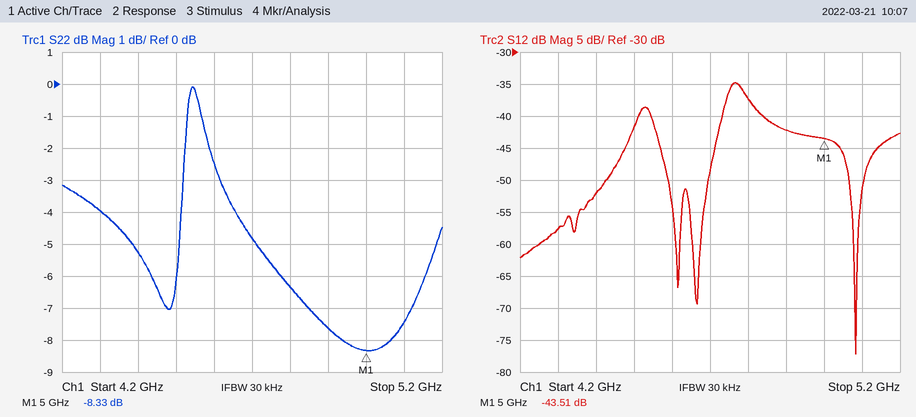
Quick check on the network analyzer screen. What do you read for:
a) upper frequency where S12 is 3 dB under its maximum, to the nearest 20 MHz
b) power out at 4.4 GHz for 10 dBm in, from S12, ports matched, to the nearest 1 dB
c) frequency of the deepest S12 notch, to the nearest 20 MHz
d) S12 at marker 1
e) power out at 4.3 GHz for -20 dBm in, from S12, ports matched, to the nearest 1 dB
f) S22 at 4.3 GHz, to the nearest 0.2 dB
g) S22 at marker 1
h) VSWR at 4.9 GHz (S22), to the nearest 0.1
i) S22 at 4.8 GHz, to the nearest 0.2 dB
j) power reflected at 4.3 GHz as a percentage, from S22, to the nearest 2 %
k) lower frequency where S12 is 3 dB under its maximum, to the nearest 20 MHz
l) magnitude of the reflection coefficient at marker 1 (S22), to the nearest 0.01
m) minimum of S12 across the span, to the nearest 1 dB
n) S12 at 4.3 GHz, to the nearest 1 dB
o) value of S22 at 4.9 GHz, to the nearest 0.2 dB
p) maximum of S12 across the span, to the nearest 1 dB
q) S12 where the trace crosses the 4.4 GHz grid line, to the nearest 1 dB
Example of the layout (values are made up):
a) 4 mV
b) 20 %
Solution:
a) 4.80 GHz
b) -42 dBm
c) 5.08 GHz
d) -43.51 dB
e) -78 dBm
f) -4.0 dB
g) -8.33 dB
h) 2.4
i) -6.4 dB
j) 40 %
k) 4.74 GHz
l) 0.38
m) -77 dB
n) -58 dB
o) -7.6 dB
p) -35 dB
q) -52 dB
